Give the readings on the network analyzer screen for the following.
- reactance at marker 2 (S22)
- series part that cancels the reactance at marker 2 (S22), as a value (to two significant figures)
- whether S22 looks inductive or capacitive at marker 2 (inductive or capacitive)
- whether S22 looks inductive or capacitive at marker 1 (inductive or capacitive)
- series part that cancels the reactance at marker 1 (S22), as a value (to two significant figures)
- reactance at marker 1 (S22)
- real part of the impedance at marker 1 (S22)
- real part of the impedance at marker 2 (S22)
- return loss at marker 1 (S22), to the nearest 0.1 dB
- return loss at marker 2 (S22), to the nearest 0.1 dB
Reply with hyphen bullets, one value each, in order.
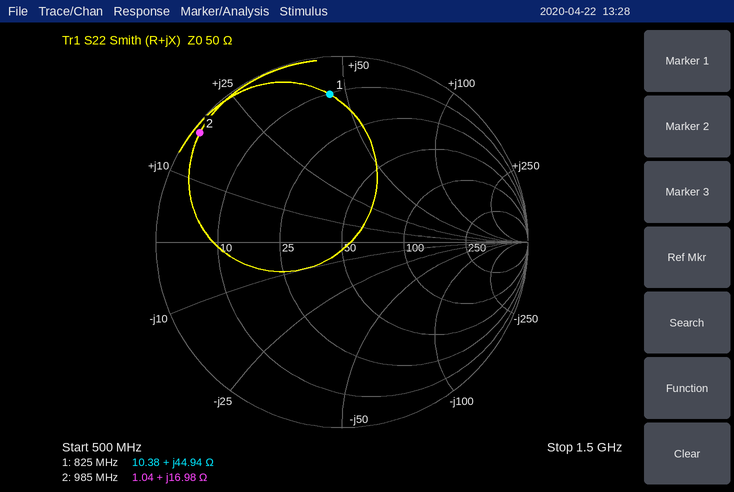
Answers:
- +16.98 Ω
- 9.5 pF
- inductive
- inductive
- 4.3 pF
- +44.94 Ω
- 10.38 Ω
- 1.04 Ω
- 2.0 dB
- 0.3 dB
